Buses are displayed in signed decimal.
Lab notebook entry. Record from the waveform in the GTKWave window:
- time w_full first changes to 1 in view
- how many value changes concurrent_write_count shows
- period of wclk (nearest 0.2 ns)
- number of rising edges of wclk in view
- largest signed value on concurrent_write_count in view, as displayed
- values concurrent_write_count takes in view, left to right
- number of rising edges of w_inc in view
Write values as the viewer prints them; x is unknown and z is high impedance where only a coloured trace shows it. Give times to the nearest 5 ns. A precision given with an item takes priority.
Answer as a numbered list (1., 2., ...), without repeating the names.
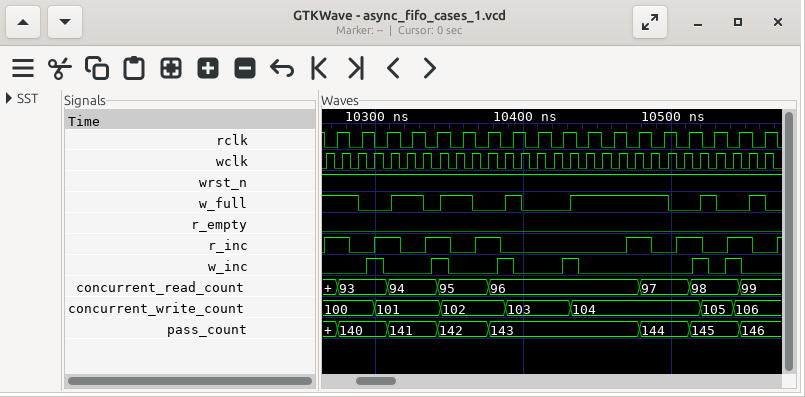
1. 10310 ns
2. 6
3. 11 ns
4. 28
5. 106
6. 100, 101, 102, 103, 104, 105, 106
7. 6
